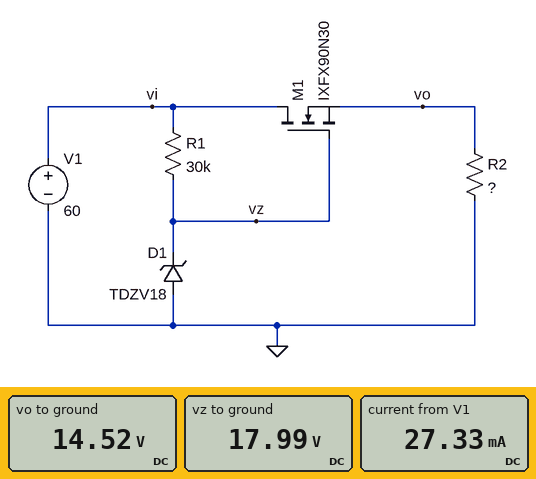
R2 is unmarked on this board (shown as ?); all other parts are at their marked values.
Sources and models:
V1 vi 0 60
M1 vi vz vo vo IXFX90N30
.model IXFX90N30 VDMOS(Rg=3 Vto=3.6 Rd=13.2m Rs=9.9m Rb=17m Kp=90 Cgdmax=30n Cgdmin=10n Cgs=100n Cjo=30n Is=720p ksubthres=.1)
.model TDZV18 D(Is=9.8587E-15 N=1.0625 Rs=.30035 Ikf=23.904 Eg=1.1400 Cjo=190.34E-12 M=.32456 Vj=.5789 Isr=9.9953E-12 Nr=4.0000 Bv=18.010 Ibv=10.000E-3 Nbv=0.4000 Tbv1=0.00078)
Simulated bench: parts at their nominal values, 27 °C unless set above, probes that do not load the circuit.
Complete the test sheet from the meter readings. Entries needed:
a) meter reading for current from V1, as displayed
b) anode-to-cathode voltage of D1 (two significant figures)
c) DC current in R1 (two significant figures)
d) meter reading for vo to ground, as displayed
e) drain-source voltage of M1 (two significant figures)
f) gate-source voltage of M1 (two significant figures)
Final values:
27.33 mA
-18 V
1.4 mA
14.52 V
45 V
3.5 V
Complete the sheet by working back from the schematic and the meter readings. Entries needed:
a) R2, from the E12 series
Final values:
560 Ω
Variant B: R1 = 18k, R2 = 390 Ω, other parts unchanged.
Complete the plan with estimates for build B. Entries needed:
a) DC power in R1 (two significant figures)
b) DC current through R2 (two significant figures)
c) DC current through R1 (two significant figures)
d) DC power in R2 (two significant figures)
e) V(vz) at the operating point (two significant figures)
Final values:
98 mW
37 mA
2.3 mA
540 mW
18 V
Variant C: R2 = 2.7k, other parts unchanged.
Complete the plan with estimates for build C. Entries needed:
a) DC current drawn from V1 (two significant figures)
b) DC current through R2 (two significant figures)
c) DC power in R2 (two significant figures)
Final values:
6.8 mA
5.4 mA
79 mW
